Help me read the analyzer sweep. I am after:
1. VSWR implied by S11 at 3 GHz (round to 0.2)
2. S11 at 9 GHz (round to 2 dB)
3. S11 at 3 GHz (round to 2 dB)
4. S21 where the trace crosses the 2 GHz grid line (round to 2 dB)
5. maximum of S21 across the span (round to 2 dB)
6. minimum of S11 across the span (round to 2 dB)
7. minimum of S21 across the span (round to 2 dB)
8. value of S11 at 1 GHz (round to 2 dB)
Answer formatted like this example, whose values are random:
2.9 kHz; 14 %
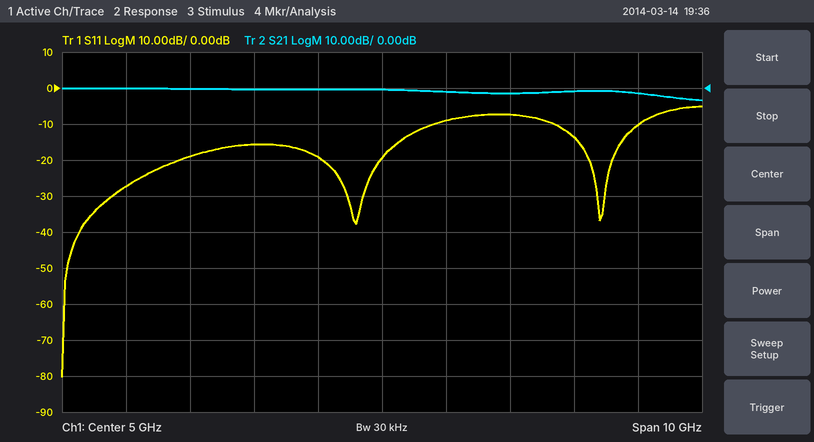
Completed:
1.4; -10 dB; -16 dB; 0 dB; 0 dB; -80 dB; -4 dB; -28 dB
